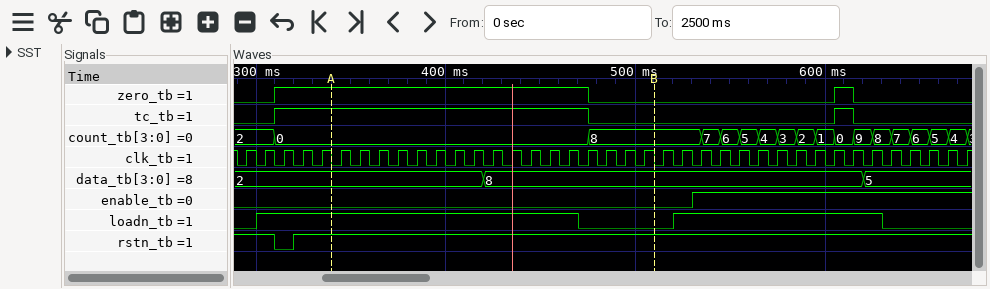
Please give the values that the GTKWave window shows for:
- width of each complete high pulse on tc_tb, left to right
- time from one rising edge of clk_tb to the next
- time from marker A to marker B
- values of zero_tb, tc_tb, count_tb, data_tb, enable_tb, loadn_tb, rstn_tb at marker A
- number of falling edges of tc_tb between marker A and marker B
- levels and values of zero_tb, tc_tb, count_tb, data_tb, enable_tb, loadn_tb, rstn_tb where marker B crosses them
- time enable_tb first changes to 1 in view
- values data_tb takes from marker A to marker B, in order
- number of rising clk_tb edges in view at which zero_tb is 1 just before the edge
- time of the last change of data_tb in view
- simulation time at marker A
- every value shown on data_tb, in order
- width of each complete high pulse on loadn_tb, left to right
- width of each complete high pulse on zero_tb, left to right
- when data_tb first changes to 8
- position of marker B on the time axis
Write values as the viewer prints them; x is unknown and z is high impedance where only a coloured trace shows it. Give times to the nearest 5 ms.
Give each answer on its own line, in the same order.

165 ms, 10 ms
10 ms
170 ms
zero_tb=1, tc_tb=1, count_tb=0, data_tb=2, enable_tb=0, loadn_tb=1, rstn_tb=1
1
zero_tb=0, tc_tb=0, count_tb=8, data_tb=8, enable_tb=0, loadn_tb=0, rstn_tb=1
530 ms
2, 8
18
620 ms
340 ms
2, 8, 5
170 ms, 110 ms
165 ms, 10 ms
420 ms
510 ms
